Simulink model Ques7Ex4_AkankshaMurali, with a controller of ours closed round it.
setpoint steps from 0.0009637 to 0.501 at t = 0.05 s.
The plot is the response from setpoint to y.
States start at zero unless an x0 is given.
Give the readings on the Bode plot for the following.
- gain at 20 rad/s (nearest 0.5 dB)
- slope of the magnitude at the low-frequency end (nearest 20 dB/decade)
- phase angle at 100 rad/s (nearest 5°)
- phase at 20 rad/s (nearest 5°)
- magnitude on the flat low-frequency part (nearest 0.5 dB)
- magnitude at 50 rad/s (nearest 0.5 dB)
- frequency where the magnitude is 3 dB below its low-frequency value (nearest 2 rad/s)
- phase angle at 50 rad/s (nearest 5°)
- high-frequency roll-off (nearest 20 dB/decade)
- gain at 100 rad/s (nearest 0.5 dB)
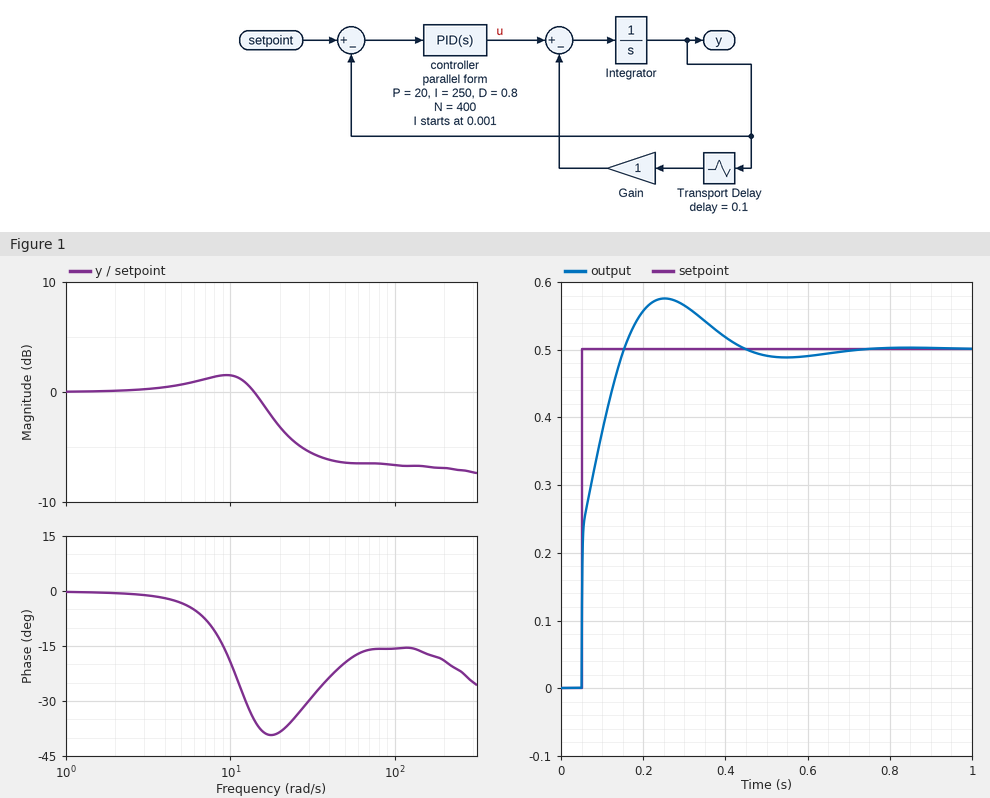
-3.0 dB
0 dB/decade
-15°
-40°
0.0 dB
-6.5 dB
20 rad/s
-20°
0 dB/decade
-6.5 dB
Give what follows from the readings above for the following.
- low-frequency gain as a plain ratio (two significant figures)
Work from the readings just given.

1.0
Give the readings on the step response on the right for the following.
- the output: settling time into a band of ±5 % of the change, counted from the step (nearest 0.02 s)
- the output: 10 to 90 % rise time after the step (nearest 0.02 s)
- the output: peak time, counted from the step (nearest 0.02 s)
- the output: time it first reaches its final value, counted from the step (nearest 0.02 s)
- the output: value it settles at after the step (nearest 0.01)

0.34 s
0.08 s
0.20 s
0.10 s
0.50
